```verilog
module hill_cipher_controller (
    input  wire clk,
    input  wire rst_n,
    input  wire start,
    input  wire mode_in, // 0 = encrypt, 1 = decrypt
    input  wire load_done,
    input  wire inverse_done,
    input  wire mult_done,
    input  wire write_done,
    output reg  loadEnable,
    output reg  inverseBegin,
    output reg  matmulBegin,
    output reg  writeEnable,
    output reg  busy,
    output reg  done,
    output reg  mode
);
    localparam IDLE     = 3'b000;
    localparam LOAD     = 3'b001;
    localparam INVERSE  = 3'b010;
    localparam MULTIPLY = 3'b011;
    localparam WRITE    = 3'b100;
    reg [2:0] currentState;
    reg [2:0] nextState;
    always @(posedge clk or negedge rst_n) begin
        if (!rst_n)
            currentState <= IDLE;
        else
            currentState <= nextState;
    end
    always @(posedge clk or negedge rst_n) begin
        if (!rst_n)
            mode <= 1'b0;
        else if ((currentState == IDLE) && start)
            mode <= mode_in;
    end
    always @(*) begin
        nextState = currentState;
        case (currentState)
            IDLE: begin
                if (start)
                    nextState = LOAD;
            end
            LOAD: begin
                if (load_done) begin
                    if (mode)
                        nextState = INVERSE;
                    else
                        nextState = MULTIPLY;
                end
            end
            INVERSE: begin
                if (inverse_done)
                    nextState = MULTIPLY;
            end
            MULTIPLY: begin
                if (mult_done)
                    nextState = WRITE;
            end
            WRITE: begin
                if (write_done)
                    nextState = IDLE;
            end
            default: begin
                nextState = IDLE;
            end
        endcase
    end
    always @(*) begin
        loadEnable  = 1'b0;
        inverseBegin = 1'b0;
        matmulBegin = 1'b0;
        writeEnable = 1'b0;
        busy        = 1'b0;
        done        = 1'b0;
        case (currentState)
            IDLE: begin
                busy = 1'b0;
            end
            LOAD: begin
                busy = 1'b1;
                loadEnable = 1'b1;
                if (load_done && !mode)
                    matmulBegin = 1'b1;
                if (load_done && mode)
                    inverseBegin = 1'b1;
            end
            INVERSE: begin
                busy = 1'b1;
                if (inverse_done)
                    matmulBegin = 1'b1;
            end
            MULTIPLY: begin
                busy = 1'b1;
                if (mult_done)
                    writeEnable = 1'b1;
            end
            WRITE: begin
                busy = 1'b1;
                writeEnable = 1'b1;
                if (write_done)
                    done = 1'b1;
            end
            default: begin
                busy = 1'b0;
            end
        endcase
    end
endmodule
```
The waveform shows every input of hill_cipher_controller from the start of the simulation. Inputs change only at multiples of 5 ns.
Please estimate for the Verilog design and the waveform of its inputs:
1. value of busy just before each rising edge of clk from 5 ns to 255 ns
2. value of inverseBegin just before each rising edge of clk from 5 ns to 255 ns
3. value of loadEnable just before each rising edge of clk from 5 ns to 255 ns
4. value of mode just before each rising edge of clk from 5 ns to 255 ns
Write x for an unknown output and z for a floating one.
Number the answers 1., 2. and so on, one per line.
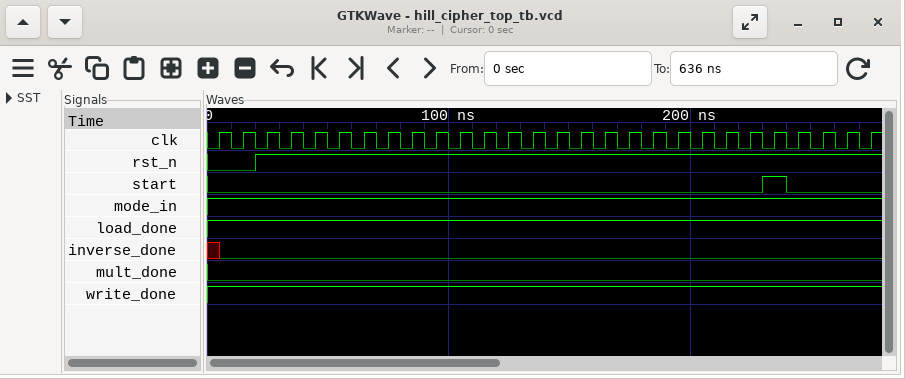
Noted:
1. 0 0 0 0 0 0 0 0 0 0 0 0 0 0 0 0 0 0 0 0 0 0 0 0 1 1
2. 0 0 0 0 0 0 0 0 0 0 0 0 0 0 0 0 0 0 0 0 0 0 0 0 1 0
3. 0 0 0 0 0 0 0 0 0 0 0 0 0 0 0 0 0 0 0 0 0 0 0 0 1 0
4. 0 0 0 0 0 0 0 0 0 0 0 0 0 0 0 0 0 0 0 0 0 0 0 0 1 1
